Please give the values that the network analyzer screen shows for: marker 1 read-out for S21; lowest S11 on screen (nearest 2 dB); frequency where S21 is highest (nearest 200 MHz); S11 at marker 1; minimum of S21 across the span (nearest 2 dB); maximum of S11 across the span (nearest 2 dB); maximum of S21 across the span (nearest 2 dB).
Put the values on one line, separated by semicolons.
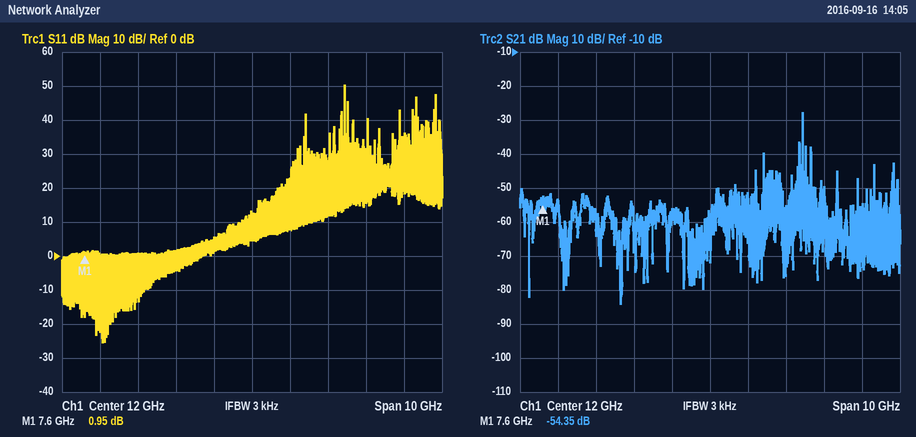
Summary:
-54.35 dB; -26 dB; 14.4 GHz; 0.95 dB; -84 dB; 50 dB; -28 dB
